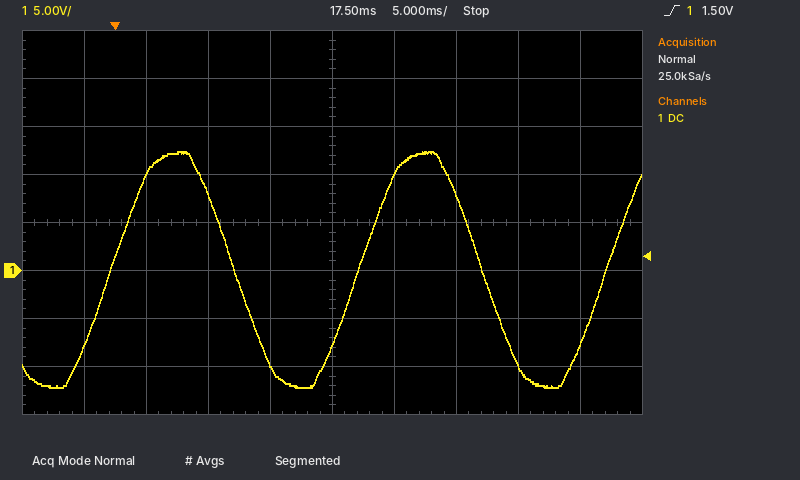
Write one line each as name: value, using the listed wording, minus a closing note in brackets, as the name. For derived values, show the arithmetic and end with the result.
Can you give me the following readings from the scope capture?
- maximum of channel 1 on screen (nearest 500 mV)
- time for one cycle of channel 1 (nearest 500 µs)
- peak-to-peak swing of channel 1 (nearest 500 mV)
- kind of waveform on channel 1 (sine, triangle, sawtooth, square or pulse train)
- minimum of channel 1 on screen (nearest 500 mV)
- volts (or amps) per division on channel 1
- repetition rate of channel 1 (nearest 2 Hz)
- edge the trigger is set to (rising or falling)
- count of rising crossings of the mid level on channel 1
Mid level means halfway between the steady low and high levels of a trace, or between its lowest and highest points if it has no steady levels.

maximum of channel 1 on screen: 12.5 V
time for one cycle of channel 1: 20.0 ms
peak-to-peak swing of channel 1: 12.5 V − (-12.0 V) = 24.5 V
kind of waveform on channel 1: sine
minimum of channel 1 on screen: -12.0 V
volts (or amps) per division on channel 1: 5 V
repetition rate of channel 1: 1 / 20.0 ms ≈ 50 Hz
edge the trigger is set to: rising
count of rising crossings of the mid level on channel 1: 3
